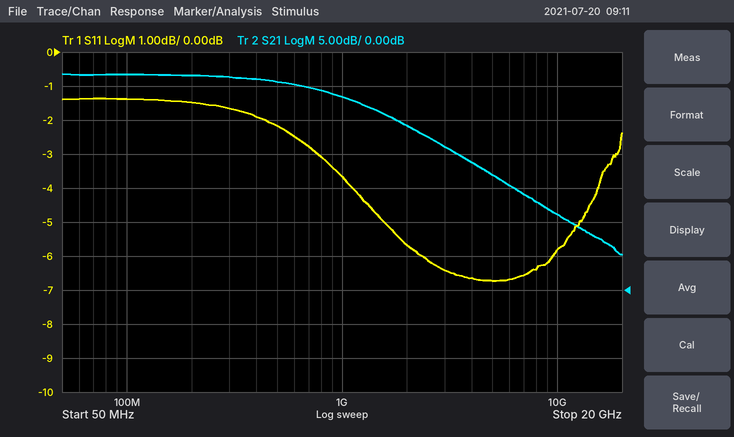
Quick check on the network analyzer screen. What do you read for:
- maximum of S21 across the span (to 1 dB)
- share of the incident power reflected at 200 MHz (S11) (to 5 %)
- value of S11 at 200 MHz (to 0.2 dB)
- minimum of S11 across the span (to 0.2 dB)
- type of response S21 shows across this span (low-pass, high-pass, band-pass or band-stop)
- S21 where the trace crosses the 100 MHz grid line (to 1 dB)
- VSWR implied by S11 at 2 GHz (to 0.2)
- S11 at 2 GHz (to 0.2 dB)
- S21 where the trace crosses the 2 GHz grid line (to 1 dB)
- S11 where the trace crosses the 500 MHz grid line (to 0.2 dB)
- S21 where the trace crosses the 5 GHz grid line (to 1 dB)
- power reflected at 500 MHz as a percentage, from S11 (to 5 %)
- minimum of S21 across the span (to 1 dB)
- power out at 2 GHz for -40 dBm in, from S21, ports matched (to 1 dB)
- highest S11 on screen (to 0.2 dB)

32 dB
70 %
-1.4 dB
-6.8 dB
low-pass
32 dB
3.2
-5.6 dB
24 dB
-2.2 dB
17 dB
60 %
5 dB
-16 dBm
-1.4 dB
